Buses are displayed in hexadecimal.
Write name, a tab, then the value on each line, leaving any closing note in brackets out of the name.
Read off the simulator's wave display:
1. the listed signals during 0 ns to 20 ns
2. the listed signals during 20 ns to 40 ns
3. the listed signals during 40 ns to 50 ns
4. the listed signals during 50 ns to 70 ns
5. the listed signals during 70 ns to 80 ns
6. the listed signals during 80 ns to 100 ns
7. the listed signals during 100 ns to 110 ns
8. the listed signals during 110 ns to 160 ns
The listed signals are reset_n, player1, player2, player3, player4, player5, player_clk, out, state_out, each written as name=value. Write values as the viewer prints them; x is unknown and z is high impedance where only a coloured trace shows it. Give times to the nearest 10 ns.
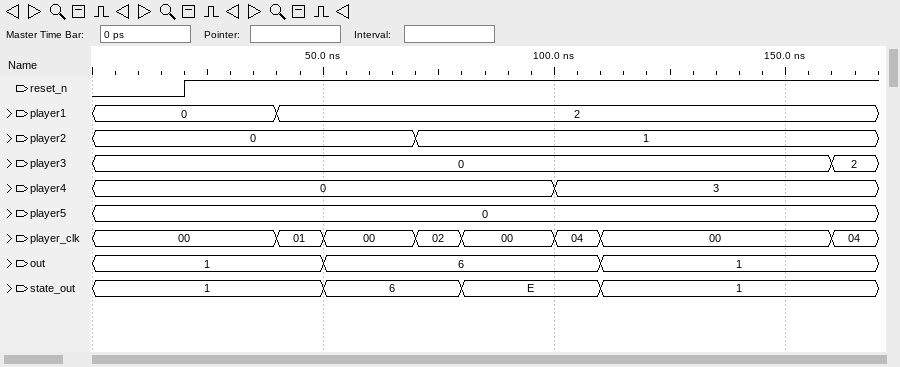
the listed signals during 0 ns to 20 ns	reset_n=0, player1=0, player2=0, player3=0, player4=0, player5=0, player_clk=00, out=1, state_out=1
the listed signals during 20 ns to 40 ns	reset_n=1, player1=0, player2=0, player3=0, player4=0, player5=0, player_clk=00, out=1, state_out=1
the listed signals during 40 ns to 50 ns	reset_n=1, player1=2, player2=0, player3=0, player4=0, player5=0, player_clk=01, out=1, state_out=1
the listed signals during 50 ns to 70 ns	reset_n=1, player1=2, player2=0, player3=0, player4=0, player5=0, player_clk=00, out=6, state_out=6
the listed signals during 70 ns to 80 ns	reset_n=1, player1=2, player2=1, player3=0, player4=0, player5=0, player_clk=02, out=6, state_out=6
the listed signals during 80 ns to 100 ns	reset_n=1, player1=2, player2=1, player3=0, player4=0, player5=0, player_clk=00, out=6, state_out=E
the listed signals during 100 ns to 110 ns	reset_n=1, player1=2, player2=1, player3=0, player4=3, player5=0, player_clk=04, out=6, state_out=E
the listed signals during 110 ns to 160 ns	reset_n=1, player1=2, player2=1, player3=0, player4=3, player5=0, player_clk=00, out=1, state_out=1
